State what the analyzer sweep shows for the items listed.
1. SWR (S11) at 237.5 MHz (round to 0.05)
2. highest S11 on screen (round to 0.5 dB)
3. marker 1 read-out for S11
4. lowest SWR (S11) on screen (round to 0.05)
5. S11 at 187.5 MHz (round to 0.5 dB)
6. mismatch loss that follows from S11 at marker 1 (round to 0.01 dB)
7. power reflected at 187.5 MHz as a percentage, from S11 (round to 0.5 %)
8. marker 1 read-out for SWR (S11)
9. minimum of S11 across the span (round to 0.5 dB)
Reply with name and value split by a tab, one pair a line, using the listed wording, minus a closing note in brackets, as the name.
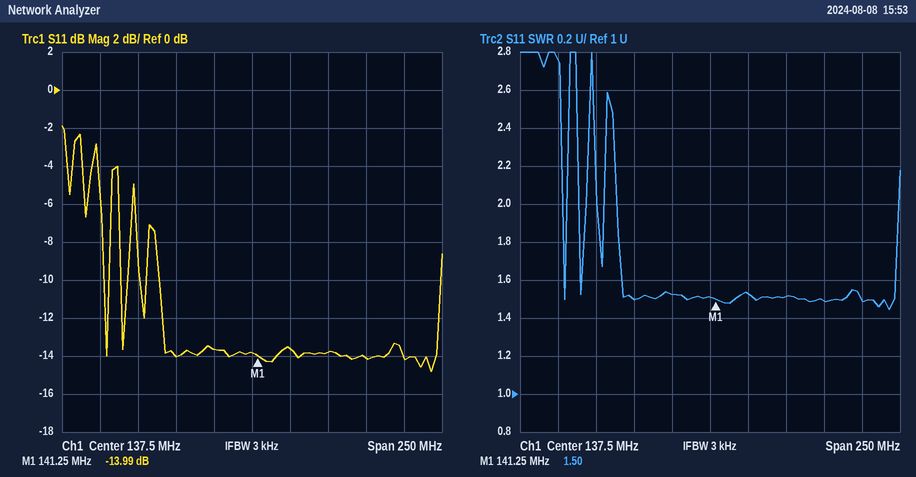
SWR (S11) at 237.5 MHz	1.50
highest S11 on screen	-2.0 dB
marker 1 read-out for S11	-13.99 dB
lowest SWR (S11) on screen	1.45
S11 at 187.5 MHz	-14.0 dB
mismatch loss that follows from S11 at marker 1	0.18 dB
power reflected at 187.5 MHz as a percentage, from S11	4.0 %
marker 1 read-out for SWR	1.50
minimum of S11 across the span	-15.0 dB
